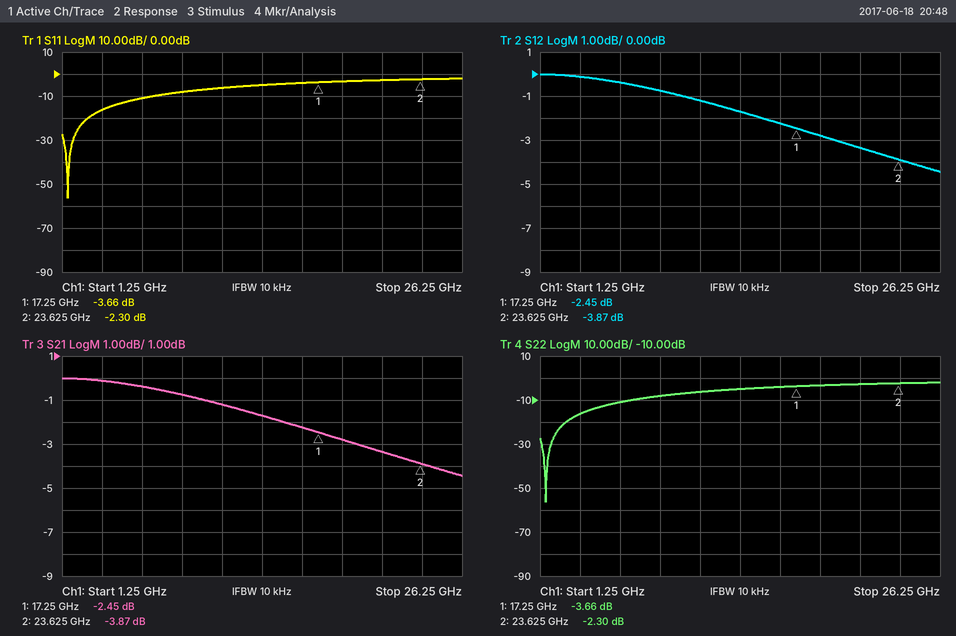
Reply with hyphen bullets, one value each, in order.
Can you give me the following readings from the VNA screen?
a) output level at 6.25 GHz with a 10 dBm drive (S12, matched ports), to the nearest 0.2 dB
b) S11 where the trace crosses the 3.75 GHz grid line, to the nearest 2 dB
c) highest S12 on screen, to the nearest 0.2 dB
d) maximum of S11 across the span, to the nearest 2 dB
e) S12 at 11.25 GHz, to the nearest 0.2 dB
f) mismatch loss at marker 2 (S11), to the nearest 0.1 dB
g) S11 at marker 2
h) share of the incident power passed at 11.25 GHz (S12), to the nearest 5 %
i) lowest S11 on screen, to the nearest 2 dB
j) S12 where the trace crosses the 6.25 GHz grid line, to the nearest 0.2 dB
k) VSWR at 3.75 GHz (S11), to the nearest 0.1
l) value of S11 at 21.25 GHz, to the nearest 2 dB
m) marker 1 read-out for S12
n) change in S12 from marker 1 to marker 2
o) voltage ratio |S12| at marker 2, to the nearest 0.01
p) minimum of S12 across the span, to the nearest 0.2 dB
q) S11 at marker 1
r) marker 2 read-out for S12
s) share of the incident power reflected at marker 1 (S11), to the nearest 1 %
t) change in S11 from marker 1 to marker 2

- 9.6 dBm
- -16 dB
- 0.0 dB
- -2 dB
- -1.2 dB
- 3.9 dB
- -2.30 dB
- 75 %
- -56 dB
- -0.4 dB
- 1.4
- -2 dB
- -2.45 dB
- -1.42 dB
- 0.64
- -4.4 dB
- -3.66 dB
- -3.87 dB
- 43 %
- 1.36 dB
